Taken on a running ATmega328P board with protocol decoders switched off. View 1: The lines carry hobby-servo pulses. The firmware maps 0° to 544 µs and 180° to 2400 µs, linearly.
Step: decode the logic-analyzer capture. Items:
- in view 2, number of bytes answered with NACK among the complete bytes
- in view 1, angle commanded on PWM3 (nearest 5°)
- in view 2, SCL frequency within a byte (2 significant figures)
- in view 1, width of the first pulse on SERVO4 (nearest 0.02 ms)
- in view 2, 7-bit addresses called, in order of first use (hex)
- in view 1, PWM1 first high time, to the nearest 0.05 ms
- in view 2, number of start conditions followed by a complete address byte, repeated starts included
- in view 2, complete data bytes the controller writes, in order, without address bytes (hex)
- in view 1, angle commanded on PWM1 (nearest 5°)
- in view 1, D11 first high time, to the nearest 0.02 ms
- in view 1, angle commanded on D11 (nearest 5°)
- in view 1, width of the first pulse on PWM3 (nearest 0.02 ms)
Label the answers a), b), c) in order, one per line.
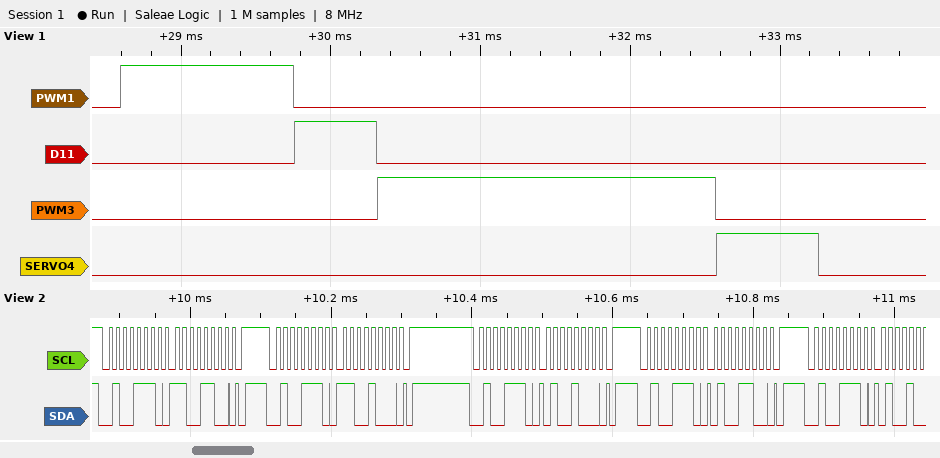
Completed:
a) 0
b) 165°
c) 100 kHz
d) 0.68 ms
e) 0x27
f) 1.15 ms
g) 5
h) CC C8 48 4C
i) 60°
j) 0.54 ms
k) 0°
l) 2.26 ms
